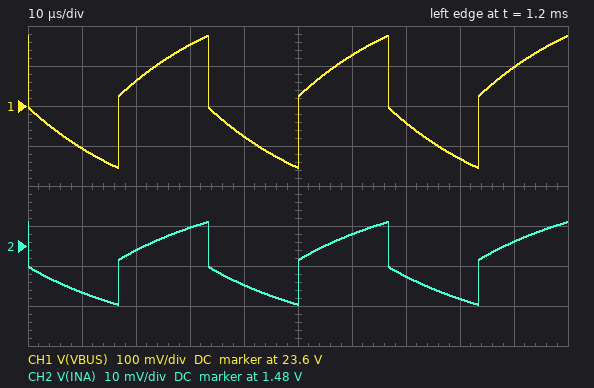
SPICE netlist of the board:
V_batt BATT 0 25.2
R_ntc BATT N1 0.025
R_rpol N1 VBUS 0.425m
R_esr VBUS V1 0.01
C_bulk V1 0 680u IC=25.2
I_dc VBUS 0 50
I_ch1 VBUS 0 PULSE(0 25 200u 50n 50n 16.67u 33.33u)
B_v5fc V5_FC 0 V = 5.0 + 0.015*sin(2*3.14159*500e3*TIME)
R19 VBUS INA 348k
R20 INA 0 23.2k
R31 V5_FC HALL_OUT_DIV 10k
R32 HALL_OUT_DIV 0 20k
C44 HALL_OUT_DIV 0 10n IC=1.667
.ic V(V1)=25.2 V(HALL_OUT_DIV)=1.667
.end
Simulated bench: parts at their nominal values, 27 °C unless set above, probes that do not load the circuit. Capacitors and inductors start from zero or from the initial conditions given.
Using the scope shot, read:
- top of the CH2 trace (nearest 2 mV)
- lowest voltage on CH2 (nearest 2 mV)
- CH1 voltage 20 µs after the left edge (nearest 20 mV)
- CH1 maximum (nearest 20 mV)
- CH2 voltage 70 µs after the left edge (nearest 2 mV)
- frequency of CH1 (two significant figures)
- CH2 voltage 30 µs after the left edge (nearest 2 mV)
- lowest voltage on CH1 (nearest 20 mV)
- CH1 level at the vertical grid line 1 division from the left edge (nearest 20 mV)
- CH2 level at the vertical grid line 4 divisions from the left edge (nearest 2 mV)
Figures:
1.486 V
1.466 V
23.66 V
23.78 V
1.472 V
30 kHz
1.484 V
23.44 V
23.50 V
1.470 V
